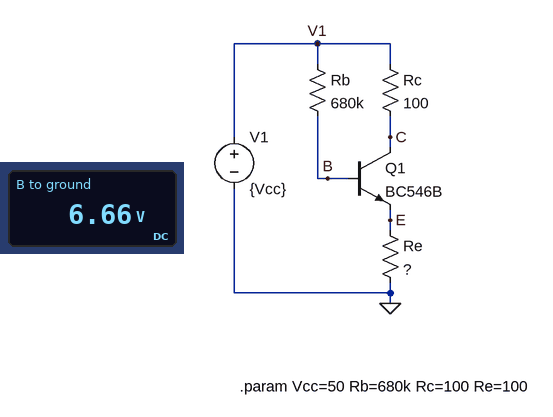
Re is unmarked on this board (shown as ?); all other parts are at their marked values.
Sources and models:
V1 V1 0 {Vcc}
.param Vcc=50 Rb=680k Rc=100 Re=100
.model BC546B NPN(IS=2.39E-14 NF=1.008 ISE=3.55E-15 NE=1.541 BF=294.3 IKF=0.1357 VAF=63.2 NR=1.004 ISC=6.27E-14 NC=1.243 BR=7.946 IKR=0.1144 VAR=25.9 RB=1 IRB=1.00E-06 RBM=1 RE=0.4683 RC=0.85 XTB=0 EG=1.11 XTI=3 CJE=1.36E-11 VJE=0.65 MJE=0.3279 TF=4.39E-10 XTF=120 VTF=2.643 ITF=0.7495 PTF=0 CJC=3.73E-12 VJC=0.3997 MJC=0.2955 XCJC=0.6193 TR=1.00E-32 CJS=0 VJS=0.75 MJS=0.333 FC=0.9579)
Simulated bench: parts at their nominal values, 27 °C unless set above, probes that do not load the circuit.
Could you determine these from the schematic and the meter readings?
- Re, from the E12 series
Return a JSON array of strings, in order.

["220 Ω"]
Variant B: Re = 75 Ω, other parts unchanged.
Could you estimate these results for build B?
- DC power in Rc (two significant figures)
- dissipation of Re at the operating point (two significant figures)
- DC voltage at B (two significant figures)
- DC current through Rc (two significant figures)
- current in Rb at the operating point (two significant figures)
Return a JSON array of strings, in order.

["89 mW", "67 mW", "3.0 V", "30 mA", "69 µA"]
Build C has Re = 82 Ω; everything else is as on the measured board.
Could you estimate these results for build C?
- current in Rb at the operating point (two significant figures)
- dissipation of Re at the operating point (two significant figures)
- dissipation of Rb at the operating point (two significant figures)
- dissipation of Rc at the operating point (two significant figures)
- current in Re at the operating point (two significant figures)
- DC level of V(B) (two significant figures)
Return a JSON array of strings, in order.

["69 µA", "73 mW", "3.2 mW", "88 mW", "30 mA", "3.2 V"]
